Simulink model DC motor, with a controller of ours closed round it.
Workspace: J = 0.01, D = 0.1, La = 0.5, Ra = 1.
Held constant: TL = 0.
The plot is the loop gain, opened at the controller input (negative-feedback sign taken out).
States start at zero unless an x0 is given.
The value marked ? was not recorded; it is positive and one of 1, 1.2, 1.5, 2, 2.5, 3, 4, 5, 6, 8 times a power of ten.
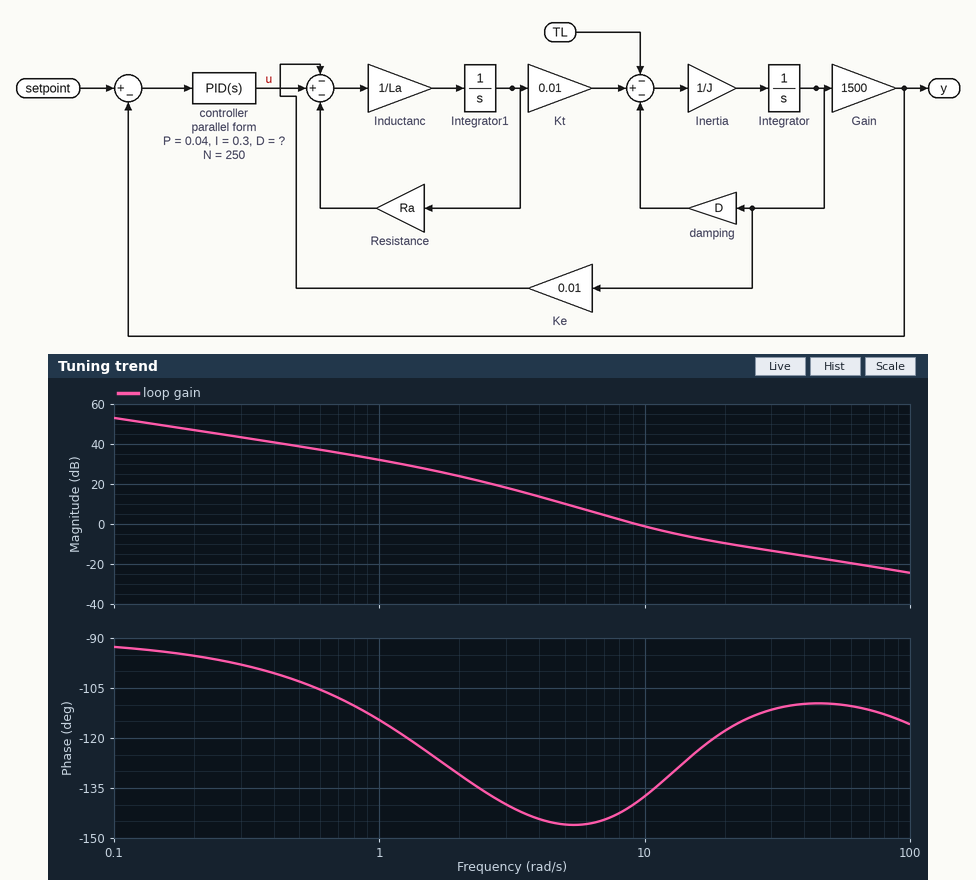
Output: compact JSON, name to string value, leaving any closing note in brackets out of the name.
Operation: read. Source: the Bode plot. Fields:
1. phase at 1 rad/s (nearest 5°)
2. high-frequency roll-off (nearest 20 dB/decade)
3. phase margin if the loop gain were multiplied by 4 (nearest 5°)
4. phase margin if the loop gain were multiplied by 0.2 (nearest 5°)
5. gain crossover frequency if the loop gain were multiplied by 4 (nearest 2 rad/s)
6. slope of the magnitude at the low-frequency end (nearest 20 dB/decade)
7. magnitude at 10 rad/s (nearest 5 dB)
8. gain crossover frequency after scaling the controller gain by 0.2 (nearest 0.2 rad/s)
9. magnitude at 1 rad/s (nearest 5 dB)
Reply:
{"phase at 1 rad/s": "-115°", "high-frequency roll-off": "-20 dB/decade", "phase margin if the loop gain were multiplied by 4": "65°", "phase margin if the loop gain were multiplied by 0.2": "35°", "gain crossover frequency if the loop gain were multiplied by 4": "26 rad/s", "slope of the magnitude at the low-frequency end": "-20 dB/decade", "magnitude at 10 rad/s": "0 dB", "gain crossover frequency after scaling the controller gain by 0.2": "4.0 rad/s", "magnitude at 1 rad/s": "30 dB"}
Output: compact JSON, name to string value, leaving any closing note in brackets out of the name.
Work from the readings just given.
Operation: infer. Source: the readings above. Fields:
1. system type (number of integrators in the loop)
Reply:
{"system type": "1"}
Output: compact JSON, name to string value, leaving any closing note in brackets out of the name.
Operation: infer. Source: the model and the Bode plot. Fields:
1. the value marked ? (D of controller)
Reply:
{"the value marked ?": "0.002"}
